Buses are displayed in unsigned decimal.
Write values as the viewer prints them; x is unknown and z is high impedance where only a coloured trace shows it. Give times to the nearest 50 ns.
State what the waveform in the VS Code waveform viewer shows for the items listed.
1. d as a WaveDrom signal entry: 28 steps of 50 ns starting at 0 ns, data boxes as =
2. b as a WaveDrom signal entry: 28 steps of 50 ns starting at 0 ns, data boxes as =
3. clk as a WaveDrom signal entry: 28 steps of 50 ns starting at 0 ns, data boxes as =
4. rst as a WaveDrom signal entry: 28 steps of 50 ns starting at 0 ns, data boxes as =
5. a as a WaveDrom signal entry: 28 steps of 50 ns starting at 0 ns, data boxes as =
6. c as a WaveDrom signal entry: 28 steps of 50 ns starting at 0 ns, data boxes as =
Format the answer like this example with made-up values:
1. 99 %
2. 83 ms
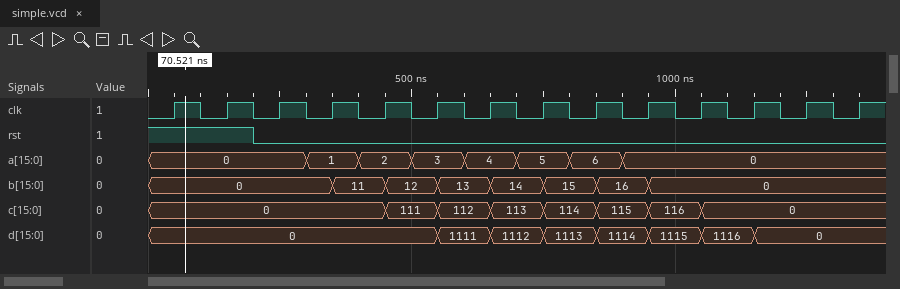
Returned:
1. {name: 'd', wave: '=..........=.=.=.=.=.=.=....', data: '0 1111 1112 1113 1114 1115 1116 0'}
2. {name: 'b', wave: '=......=.=.=.=.=.=.=........', data: '0 11 12 13 14 15 16 0'}
3. {name: 'clk', wave: '0101010101010101010101010101'}
4. {name: 'rst', wave: '1...0.......................'}
5. {name: 'a', wave: '=.....=.=.=.=.=.=.=.........', data: '0 1 2 3 4 5 6 0'}
6. {name: 'c', wave: '=........=.=.=.=.=.=.=......', data: '0 111 112 113 114 115 116 0'}
